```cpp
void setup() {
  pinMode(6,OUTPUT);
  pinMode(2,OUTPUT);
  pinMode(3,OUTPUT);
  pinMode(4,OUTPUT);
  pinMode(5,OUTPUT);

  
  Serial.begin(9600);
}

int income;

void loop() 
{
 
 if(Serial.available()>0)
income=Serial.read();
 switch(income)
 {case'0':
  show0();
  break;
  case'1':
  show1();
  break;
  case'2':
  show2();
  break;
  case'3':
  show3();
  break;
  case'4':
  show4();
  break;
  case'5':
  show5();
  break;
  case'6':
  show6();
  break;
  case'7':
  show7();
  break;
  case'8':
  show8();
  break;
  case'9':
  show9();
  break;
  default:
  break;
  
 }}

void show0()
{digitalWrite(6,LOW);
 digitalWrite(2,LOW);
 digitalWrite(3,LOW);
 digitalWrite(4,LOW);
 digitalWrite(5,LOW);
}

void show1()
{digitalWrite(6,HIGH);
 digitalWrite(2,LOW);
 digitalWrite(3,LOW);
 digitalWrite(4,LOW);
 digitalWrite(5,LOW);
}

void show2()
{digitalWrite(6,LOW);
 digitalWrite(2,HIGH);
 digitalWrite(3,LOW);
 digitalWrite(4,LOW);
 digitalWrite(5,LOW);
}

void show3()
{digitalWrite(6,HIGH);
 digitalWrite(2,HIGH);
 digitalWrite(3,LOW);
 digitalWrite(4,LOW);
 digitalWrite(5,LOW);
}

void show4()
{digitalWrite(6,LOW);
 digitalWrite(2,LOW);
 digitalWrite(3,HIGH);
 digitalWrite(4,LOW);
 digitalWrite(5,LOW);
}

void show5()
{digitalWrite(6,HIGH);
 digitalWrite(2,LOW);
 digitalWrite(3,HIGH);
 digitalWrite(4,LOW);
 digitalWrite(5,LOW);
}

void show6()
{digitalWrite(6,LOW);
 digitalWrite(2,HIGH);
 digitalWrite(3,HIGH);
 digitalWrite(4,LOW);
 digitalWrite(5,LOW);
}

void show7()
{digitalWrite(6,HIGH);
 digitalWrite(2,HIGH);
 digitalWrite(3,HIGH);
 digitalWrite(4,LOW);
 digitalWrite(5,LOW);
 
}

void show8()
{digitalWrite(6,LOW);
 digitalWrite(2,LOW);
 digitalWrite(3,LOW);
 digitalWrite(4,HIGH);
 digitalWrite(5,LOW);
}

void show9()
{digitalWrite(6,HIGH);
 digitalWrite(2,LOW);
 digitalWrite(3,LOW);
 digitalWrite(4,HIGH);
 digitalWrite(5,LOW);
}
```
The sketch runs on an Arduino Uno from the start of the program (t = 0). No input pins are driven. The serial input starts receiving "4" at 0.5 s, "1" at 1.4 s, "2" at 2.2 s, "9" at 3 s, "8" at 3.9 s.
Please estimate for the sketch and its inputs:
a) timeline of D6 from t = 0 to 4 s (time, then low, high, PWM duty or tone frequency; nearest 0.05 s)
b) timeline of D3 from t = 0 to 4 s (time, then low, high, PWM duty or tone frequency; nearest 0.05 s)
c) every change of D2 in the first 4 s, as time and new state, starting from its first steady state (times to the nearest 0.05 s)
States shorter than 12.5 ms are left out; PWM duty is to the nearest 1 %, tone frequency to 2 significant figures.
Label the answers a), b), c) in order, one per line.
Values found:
a) 0 s low; 1.4 s high; 2.2 s low; 3 s high; 3.9 s low
b) 0 s low; 0.5 s high; 1.4 s low
c) 0 s low; 2.2 s high; 3 s low
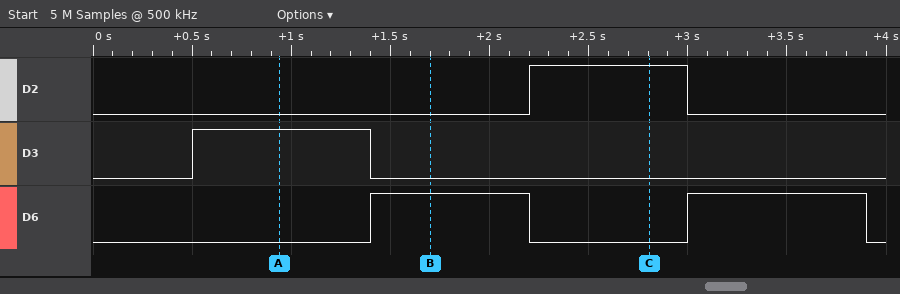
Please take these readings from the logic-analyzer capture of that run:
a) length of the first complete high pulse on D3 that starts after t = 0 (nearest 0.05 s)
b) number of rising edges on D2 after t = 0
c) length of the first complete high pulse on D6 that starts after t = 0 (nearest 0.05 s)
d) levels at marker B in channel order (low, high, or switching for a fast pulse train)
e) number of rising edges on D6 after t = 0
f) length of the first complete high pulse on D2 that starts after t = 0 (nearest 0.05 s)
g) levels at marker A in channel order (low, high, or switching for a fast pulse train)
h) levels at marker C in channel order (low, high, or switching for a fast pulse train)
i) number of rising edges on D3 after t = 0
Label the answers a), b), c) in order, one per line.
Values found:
a) 0.90 s
b) 1
c) 0.80 s
d) D2 low, D3 low, D6 high
e) 2
f) 0.80 s
g) D2 low, D3 high, D6 low
h) D2 high, D3 low, D6 low
i) 1
